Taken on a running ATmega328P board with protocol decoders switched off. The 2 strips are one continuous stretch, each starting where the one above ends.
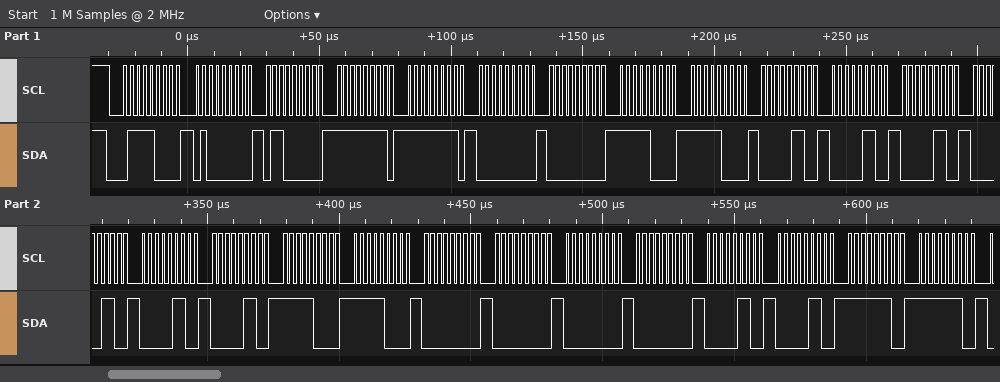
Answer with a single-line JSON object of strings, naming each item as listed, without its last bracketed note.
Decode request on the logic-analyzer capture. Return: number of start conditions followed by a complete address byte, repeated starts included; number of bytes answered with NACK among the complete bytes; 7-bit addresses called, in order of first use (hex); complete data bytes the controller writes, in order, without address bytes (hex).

{"number of start conditions followed by a complete address byte, repeated starts included": "1", "number of bytes answered with NACK among the complete bytes": "0", "7-bit addresses called, in order of first use": "0x3C", "complete data bytes the controller writes, in order, without address bytes": "40 60 FF FF 00 00 F8 F8 06 06 06 06 06 06 F8 F8 00 00 00 00 06 06 FE FE"}
